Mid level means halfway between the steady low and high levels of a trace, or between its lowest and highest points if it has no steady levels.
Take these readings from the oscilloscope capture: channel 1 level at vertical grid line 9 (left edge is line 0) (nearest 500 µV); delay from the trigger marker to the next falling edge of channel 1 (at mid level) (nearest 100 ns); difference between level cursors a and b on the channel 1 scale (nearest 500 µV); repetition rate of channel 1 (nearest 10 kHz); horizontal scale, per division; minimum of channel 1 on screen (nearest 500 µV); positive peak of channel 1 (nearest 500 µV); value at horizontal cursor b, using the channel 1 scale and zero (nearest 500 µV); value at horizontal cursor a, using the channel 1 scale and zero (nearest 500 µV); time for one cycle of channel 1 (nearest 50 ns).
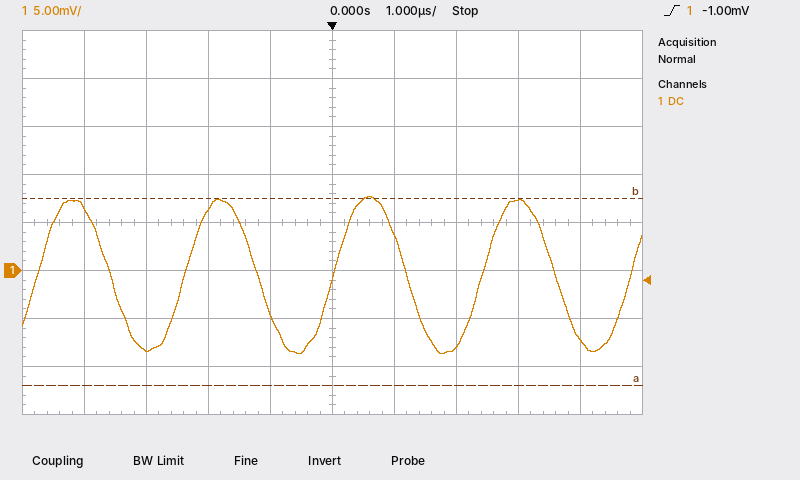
-7.0 mV
1.2 µs
19.5 mV
420 kHz
1 µs
-8.5 mV
7.5 mV
7.5 mV
-12.0 mV
2.40 µs
